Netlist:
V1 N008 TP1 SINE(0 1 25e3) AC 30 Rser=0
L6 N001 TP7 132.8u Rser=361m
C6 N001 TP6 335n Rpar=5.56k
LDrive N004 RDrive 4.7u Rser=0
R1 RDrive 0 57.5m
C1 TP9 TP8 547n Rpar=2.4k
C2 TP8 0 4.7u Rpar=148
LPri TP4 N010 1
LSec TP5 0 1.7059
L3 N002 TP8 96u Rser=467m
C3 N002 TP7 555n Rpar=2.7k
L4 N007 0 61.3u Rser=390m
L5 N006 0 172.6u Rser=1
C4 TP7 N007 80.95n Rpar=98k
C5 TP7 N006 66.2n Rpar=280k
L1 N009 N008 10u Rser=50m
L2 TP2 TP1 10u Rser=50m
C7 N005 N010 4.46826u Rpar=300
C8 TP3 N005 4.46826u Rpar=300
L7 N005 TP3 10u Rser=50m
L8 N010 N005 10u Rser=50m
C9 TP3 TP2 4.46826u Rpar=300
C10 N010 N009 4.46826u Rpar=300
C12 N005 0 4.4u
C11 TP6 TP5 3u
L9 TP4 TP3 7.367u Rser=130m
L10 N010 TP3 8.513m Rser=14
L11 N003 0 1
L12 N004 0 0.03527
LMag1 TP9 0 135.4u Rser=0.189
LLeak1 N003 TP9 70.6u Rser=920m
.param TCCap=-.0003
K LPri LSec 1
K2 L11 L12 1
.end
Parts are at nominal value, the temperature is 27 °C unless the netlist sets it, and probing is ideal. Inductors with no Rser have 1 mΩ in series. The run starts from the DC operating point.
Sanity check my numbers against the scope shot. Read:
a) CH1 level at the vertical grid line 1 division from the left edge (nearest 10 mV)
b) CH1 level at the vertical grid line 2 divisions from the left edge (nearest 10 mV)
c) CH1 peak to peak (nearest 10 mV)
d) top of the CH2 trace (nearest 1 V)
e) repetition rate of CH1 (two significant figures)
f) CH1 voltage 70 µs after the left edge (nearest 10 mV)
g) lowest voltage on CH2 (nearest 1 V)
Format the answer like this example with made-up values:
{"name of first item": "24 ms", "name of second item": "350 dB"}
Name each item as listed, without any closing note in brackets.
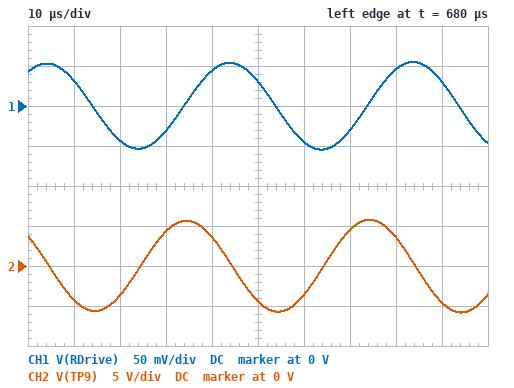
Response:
{"CH1 level at the vertical grid line 1 division from the left edge": "30 mV", "CH1 level at the vertical grid line 2 divisions from the left edge": "-40 mV", "CH1 peak to peak": "110 mV", "top of the CH2 trace": "6 V", "repetition rate of CH1": "25 kHz", "CH1 voltage 70 µs after the left edge": "-30 mV", "lowest voltage on CH2": "-6 V"}
